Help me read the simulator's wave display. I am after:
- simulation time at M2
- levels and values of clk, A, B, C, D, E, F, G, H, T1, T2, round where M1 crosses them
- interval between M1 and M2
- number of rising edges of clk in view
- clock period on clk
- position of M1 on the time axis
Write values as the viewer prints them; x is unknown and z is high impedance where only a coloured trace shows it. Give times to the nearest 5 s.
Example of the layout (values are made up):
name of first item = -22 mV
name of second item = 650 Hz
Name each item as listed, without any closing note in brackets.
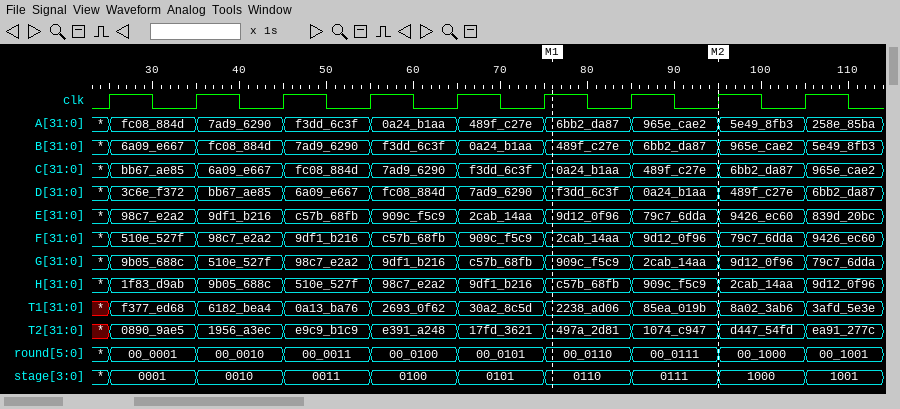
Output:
simulation time at M2 = 95 s
levels and values of clk, A, B, C, D, E, F, G, H, T1, T2, round where M1 crosses them = clk=1, A=6bb2_da87, B=489f_c27e, C=0a24_b1aa, D=f3dd_6c3f, E=9d12_0f96, F=2cab_14aa, G=909c_f5c9, H=c57b_68fb, T1=2238_ad06, T2=497a_2d81, round=00_0110
interval between M1 and M2 = 20 s
number of rising edges of clk in view = 9
clock period on clk = 10 s
position of M1 on the time axis = 75 s
